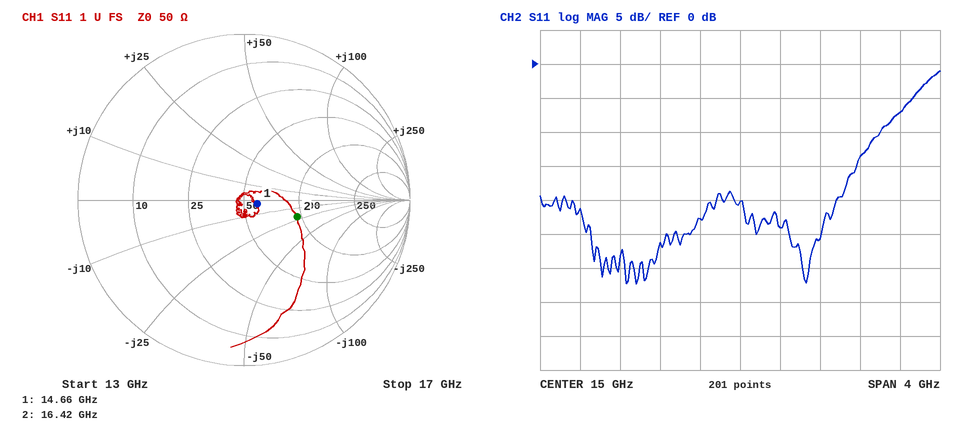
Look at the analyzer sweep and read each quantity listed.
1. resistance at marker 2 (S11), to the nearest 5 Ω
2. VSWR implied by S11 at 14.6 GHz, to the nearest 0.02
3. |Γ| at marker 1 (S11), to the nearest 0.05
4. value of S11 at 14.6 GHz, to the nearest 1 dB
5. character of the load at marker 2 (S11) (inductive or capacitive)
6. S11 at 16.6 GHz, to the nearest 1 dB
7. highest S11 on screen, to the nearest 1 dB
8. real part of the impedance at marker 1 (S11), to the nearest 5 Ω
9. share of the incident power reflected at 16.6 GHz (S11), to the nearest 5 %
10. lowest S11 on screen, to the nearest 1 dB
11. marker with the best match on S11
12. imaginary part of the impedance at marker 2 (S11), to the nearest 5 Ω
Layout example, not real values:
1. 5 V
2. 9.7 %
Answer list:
1. 95 Ω
2. 1.16
3. 0.10
4. -23 dB
5. capacitive
6. -7 dB
7. -1 dB
8. 60 Ω
9. 20 %
10. -32 dB
11. marker 1
12. -20 Ω
